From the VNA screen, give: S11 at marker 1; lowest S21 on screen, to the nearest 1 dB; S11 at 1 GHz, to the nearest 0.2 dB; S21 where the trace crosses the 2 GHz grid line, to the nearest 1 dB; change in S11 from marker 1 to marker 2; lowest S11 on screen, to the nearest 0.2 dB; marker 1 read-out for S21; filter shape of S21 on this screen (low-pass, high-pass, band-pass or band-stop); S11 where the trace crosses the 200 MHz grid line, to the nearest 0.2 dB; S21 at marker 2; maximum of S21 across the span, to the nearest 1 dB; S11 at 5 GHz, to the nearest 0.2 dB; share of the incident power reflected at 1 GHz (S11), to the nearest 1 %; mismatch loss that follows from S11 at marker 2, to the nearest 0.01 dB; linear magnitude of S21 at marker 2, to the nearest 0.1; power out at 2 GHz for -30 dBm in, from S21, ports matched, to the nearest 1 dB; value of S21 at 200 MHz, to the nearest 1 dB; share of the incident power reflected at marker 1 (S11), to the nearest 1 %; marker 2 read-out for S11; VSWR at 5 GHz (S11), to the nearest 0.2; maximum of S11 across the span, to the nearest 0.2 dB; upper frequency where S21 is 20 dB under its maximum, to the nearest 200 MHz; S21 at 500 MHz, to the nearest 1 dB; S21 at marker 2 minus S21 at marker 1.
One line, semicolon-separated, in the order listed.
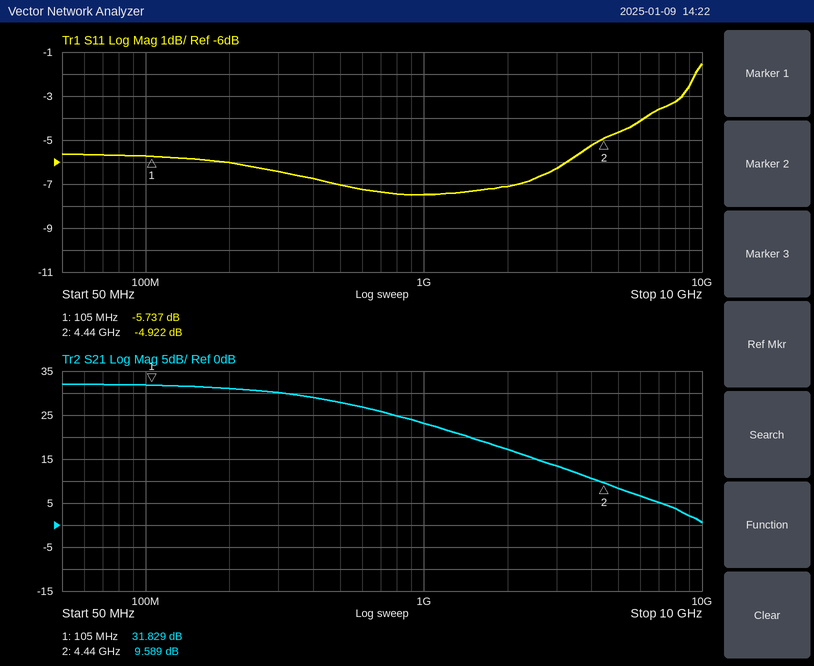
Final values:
-5.737 dB; 1 dB; -7.4 dB; 17 dB; 0.815 dB; -7.4 dB; 31.829 dB; low-pass; -6.0 dB; 9.589 dB; 32 dB; -4.6 dB; 18 %; 1.69 dB; 3.0; -13 dBm; 31 dB; 27 %; -4.922 dB; 3.8; -1.6 dB; 3.4 GHz; 28 dB; -22.240 dB
